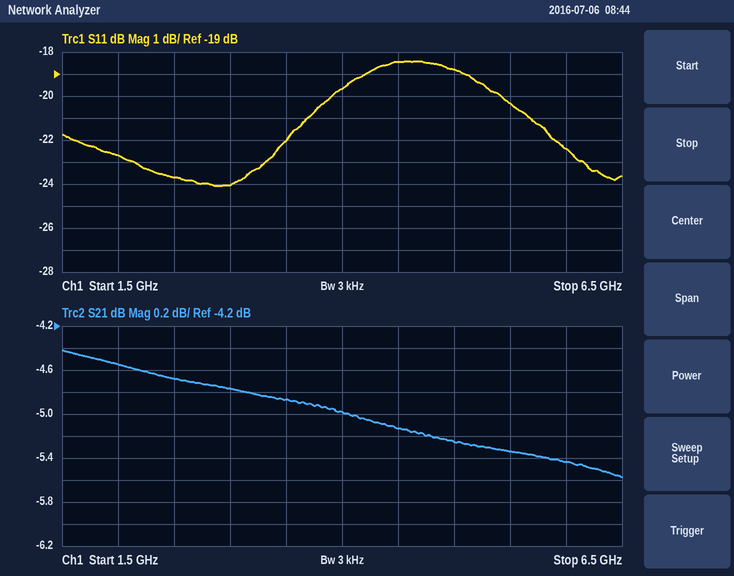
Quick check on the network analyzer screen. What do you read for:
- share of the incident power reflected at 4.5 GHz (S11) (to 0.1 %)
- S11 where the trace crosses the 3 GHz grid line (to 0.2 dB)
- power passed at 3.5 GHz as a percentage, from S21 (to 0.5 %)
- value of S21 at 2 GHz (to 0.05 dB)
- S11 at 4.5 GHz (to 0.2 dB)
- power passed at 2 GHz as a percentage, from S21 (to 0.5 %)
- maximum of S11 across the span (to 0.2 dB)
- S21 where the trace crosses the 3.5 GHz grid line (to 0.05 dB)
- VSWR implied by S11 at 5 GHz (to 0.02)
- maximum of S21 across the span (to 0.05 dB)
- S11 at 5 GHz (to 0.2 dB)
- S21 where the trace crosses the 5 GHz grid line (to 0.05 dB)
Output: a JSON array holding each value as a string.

["1.4 %", "-24.0 dB", "32.5 %", "-4.55 dB", "-18.4 dB", "35.0 %", "-18.4 dB", "-4.85 dB", "1.26", "-4.40 dB", "-18.8 dB", "-5.25 dB"]
